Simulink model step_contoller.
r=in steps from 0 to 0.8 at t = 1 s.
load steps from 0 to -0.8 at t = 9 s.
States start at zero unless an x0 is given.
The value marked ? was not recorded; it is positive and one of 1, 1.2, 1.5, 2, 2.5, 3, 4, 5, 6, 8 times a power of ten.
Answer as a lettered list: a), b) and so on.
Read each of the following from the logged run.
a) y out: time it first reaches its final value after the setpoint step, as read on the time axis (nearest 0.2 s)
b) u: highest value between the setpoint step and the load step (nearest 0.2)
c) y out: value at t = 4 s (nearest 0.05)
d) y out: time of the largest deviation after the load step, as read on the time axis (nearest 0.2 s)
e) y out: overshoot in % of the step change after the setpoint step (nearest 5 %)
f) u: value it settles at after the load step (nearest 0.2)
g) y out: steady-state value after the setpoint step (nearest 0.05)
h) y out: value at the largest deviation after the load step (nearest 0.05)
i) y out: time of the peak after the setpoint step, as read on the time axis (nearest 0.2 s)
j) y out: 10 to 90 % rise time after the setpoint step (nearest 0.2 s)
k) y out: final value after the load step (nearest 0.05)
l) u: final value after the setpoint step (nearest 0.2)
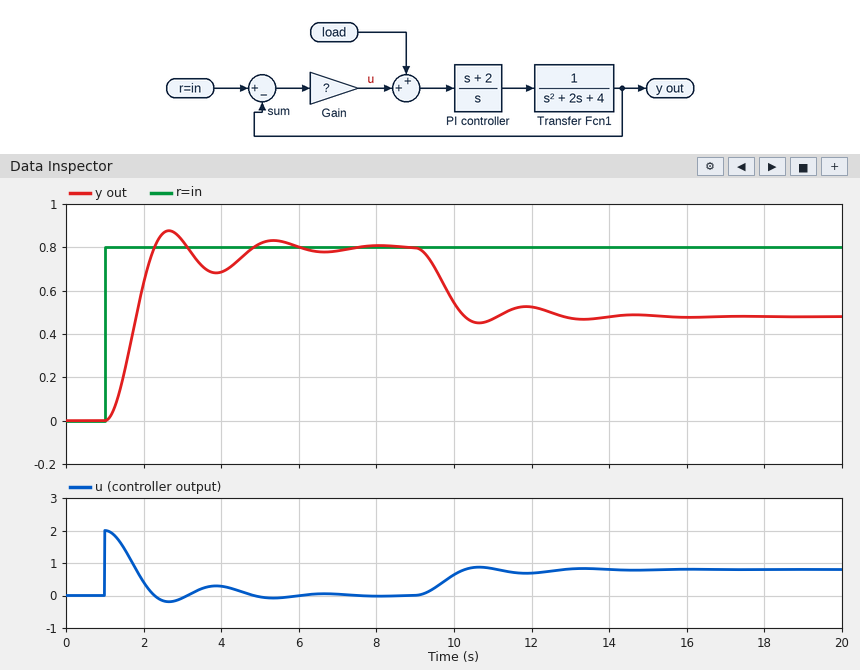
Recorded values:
a) 2.2 s
b) 2.0
c) 0.70
d) 10.6 s
e) 10 %
f) 0.8
g) 0.80
h) 0.45
i) 2.6 s
j) 0.8 s
k) 0.50
l) 0.0
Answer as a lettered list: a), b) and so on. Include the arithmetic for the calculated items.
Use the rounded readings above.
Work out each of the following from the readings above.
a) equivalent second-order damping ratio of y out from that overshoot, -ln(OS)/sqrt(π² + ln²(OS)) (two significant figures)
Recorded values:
a) ln(0.1) = -2.303; 2.303 / sqrt(9.870 + 5.302) = 0.59
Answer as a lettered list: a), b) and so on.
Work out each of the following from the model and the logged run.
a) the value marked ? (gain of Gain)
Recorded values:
a) 2.5
